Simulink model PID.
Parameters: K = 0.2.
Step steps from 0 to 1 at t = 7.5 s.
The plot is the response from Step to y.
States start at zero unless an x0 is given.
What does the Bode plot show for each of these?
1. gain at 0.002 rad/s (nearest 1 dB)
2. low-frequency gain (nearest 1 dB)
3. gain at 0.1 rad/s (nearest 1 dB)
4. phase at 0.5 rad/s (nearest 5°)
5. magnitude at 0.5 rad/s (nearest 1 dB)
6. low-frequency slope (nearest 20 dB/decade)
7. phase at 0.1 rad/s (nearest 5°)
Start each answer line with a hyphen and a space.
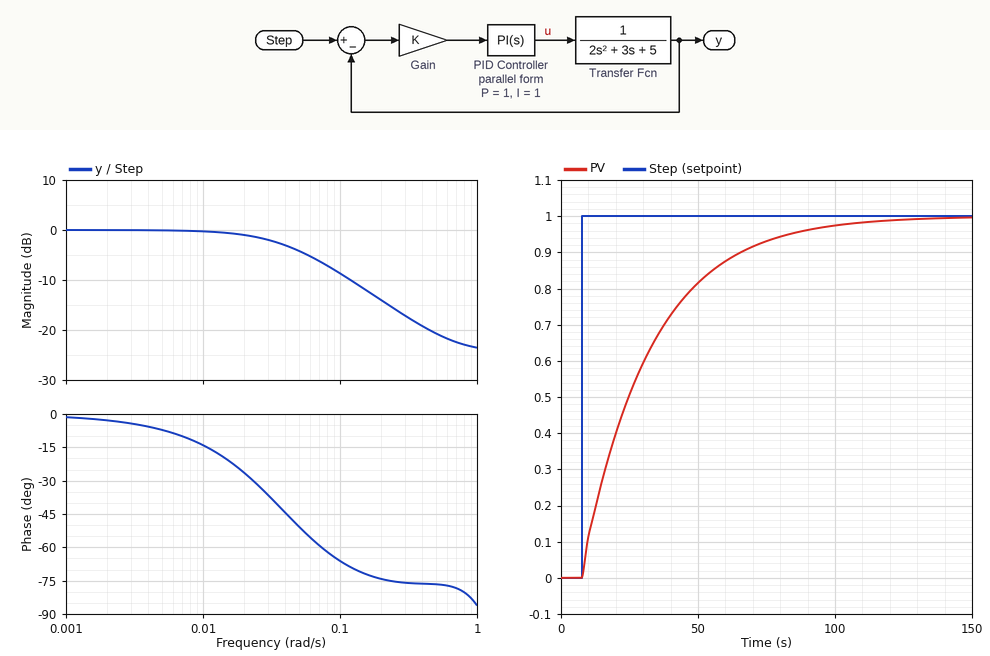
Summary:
- 0 dB
- 0 dB
- -9 dB
- -75°
- -21 dB
- 0 dB/decade
- -65°
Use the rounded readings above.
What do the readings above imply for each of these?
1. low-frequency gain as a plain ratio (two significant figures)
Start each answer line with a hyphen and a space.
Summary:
- 1.0
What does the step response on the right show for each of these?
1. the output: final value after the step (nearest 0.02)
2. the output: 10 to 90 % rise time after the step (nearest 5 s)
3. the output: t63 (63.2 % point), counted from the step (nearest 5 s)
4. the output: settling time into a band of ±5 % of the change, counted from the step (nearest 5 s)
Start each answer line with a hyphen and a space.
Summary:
- 1.00
- 55 s
- 25 s
- 75 s
